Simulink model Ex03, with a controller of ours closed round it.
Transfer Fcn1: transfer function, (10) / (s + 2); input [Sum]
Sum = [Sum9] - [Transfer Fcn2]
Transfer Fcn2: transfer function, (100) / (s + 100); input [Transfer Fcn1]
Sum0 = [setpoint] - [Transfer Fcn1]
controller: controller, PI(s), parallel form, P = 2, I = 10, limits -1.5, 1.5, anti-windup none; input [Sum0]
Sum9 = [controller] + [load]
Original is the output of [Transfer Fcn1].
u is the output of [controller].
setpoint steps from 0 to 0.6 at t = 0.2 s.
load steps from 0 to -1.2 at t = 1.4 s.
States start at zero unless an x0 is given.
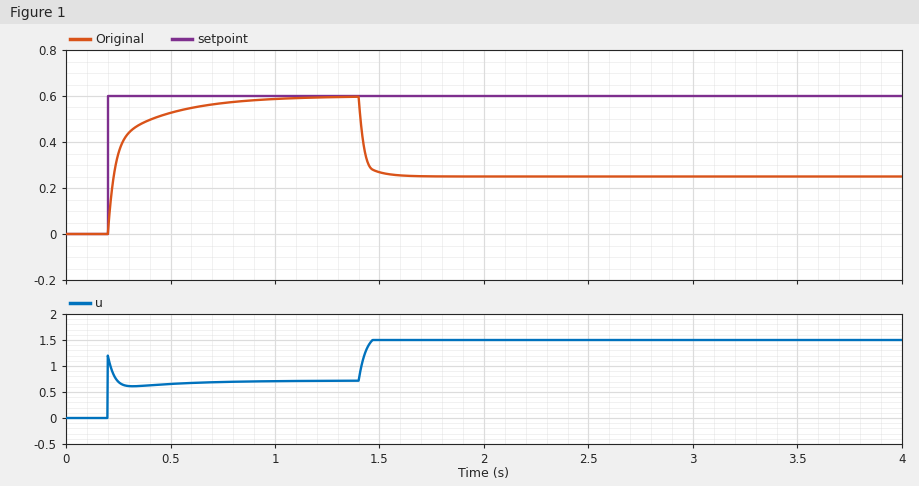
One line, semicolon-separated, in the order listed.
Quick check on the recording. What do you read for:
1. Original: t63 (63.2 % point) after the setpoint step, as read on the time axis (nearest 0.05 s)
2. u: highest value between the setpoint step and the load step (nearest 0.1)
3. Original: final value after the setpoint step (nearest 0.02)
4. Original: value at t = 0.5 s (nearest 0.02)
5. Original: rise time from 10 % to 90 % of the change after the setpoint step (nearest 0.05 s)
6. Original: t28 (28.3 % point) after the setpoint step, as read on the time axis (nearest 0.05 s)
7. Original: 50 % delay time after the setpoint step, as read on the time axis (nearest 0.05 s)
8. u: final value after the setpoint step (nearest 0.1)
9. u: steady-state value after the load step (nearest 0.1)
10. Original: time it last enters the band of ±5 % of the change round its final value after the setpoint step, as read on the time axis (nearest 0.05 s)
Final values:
0.25 s; 1.2; 0.60; 0.52; 0.35 s; 0.20 s; 0.25 s; 0.7; 1.5; 0.75 s
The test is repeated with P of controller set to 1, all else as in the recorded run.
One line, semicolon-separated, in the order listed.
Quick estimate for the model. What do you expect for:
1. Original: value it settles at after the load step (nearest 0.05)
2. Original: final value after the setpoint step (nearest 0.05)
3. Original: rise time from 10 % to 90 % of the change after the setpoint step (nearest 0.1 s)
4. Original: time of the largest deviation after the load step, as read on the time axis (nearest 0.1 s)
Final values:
0.25; 0.60; 0.3 s; 1.5 s
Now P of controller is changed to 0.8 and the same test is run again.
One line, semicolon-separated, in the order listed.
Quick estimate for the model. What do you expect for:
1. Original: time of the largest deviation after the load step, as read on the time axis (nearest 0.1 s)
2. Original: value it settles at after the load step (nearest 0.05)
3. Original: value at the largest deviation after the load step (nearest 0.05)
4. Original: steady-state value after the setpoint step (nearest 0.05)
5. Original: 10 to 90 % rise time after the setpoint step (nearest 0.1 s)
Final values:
1.5 s; 0.25; 0.15; 0.60; 0.3 s
